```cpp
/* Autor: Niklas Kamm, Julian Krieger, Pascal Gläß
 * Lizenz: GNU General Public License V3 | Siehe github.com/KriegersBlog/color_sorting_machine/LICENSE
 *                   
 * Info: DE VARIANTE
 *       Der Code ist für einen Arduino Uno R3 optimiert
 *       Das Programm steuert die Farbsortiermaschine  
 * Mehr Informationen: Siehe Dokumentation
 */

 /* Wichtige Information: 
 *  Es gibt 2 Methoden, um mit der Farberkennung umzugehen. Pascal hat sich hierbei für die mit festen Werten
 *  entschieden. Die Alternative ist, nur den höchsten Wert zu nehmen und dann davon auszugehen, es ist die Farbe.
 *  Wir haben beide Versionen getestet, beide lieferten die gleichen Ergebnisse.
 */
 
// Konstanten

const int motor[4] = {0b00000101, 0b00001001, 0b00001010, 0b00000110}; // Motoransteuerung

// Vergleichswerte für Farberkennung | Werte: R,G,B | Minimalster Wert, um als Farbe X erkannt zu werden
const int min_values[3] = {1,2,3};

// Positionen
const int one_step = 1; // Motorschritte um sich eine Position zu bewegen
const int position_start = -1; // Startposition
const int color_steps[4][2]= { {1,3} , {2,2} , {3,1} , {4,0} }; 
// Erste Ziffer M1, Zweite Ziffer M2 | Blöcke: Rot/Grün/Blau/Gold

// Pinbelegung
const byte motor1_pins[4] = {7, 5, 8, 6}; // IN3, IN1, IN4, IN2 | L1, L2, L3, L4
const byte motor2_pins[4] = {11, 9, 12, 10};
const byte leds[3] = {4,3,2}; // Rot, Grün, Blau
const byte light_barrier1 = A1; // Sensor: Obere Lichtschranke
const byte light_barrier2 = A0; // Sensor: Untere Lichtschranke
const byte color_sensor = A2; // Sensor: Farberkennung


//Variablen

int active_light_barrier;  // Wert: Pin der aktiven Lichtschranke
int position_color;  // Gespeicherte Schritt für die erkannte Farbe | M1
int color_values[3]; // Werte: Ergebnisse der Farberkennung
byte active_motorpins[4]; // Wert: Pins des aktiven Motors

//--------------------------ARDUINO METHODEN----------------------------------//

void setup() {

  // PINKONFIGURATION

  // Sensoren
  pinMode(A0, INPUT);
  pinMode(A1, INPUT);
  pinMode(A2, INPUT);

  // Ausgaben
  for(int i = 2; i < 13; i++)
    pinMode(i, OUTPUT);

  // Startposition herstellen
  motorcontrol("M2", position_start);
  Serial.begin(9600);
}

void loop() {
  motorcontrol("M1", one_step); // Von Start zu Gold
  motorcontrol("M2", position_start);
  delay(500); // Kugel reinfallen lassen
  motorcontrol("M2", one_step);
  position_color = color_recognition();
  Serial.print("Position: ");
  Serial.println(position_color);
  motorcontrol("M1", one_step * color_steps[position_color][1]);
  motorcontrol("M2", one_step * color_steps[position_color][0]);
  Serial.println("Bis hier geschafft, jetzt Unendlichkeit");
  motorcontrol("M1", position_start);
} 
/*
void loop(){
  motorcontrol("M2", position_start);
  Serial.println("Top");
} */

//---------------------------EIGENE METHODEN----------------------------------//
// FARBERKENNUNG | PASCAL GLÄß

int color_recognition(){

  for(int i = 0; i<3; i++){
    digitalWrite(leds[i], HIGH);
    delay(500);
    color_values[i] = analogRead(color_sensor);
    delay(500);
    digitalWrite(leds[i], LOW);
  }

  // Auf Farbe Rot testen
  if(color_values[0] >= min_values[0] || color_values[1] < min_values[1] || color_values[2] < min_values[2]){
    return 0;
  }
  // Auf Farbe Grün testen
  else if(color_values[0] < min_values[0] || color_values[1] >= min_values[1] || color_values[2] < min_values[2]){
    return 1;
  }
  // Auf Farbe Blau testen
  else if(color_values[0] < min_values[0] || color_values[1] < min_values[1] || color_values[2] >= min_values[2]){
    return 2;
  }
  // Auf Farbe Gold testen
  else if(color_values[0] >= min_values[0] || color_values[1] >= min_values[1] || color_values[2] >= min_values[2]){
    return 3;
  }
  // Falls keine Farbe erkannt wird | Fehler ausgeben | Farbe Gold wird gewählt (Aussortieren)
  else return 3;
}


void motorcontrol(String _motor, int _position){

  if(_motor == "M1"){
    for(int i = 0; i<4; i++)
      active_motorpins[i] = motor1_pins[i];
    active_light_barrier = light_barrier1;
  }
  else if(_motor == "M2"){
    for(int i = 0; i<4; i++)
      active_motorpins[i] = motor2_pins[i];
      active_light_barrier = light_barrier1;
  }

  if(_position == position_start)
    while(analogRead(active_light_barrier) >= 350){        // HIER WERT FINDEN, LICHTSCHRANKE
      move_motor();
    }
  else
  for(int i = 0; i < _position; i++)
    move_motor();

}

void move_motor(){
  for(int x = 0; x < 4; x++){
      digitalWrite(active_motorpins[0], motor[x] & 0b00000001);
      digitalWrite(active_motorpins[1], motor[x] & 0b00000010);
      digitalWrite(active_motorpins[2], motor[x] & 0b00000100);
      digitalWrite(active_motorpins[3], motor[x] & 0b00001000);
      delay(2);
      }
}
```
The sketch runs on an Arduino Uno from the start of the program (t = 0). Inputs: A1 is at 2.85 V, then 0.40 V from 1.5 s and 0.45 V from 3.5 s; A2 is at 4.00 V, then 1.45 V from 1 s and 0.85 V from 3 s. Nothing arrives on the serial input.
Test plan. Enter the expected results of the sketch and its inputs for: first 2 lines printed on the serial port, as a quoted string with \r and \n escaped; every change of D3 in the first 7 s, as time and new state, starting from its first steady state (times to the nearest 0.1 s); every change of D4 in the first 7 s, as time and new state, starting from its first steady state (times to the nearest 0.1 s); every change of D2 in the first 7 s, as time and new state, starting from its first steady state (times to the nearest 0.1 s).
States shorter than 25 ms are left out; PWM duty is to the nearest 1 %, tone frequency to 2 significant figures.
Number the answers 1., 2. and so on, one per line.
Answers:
1. "Position: 0\r\nBis hier geschafft, jetzt Unendlichkeit\r\n"
2. 0 s low; 3 s high; 4 s low; 6.6 s high
3. 0 s low; 2 s high; 3 s low; 5.6 s high; 6.6 s low
4. 0 s low; 4 s high; 5 s low
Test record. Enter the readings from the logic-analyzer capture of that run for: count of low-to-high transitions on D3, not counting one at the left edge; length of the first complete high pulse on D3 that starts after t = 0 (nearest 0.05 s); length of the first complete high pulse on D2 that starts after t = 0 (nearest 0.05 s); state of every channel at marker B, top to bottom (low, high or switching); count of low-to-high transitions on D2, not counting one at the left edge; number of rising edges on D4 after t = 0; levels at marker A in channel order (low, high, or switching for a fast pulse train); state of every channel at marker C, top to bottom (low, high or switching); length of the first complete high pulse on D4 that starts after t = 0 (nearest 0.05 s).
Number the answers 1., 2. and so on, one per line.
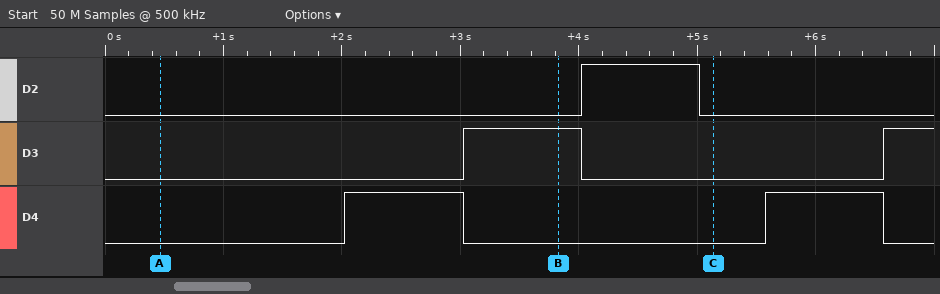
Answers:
1. 2
2. 1.00 s
3. 1.00 s
4. D2 low, D3 high, D4 low
5. 1
6. 2
7. D2 low, D3 low, D4 low
8. D2 low, D3 low, D4 low
9. 1.00 s
